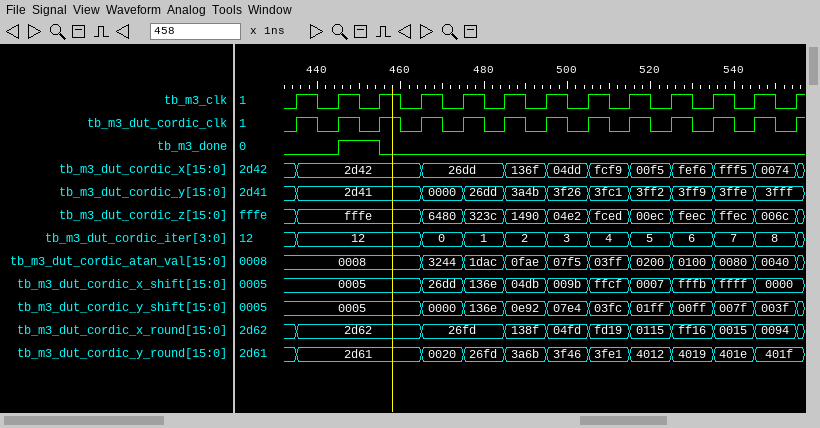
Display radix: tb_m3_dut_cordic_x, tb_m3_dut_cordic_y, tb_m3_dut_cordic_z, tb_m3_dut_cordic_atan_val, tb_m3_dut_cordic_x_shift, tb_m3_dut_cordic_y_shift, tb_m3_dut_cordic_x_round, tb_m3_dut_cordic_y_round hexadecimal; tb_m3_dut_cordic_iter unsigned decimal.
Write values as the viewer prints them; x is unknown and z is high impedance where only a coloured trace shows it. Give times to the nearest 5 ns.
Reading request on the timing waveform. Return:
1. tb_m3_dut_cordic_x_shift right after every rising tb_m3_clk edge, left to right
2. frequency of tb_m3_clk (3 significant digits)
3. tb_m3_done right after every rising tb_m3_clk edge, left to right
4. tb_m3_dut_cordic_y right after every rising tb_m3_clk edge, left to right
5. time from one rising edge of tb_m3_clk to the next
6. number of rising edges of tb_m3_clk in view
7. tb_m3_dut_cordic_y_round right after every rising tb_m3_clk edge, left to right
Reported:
0005, 0005, 0005, 26dd, 136e, 04db, 009b, ffcf, 0007, fffb, ffff, 0000, 0000
100 MHz
0 1 0 0 0 0 0 0 0 0 0 0 0
2d41, 2d41, 2d41, 0000, 26dd, 3a4b, 3f26, 3fc1, 3ff2, 3ff9, 3ffe, 3fff, 3fff
10 ns
13
2d61, 2d61, 2d61, 0020, 26fd, 3a6b, 3f46, 3fe1, 4012, 4019, 401e, 401f, 401f
